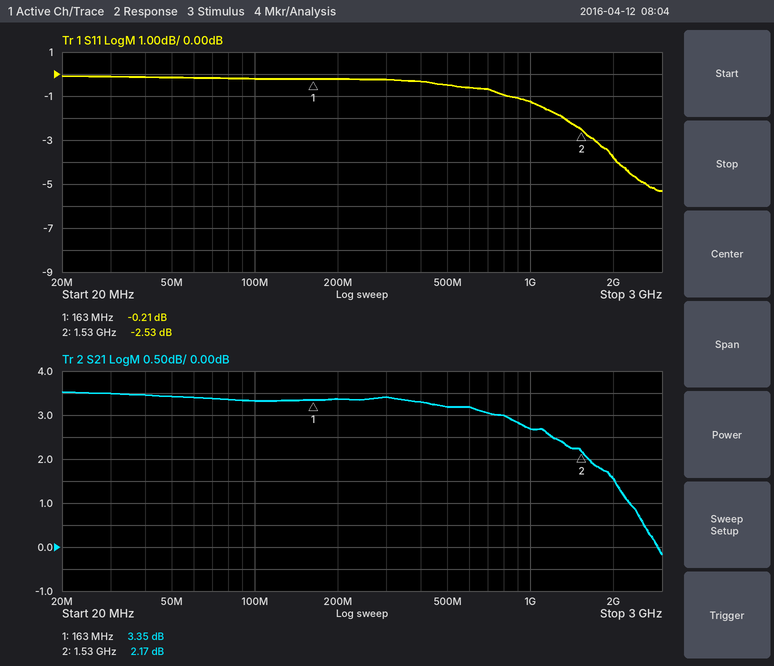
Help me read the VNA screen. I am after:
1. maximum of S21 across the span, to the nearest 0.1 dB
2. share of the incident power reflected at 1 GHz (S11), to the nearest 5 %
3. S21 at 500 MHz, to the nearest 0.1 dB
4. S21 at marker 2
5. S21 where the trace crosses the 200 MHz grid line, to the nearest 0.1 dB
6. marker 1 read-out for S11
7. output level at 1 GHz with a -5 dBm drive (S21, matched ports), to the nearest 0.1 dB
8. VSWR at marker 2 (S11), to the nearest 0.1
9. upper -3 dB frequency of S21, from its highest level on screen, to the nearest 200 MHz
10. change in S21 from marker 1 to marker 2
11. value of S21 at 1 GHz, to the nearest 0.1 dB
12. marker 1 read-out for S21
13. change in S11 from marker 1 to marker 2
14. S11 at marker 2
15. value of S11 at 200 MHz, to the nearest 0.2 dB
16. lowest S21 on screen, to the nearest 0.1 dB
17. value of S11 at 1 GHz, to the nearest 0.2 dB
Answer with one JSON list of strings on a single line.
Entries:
["3.5 dB", "75 %", "3.2 dB", "2.17 dB", "3.4 dB", "-0.21 dB", "-2.3 dBm", "6.9", "2.6 GHz", "-1.18 dB", "2.7 dB", "3.35 dB", "-2.32 dB", "-2.53 dB", "-0.2 dB", "-0.2 dB", "-1.2 dB"]
